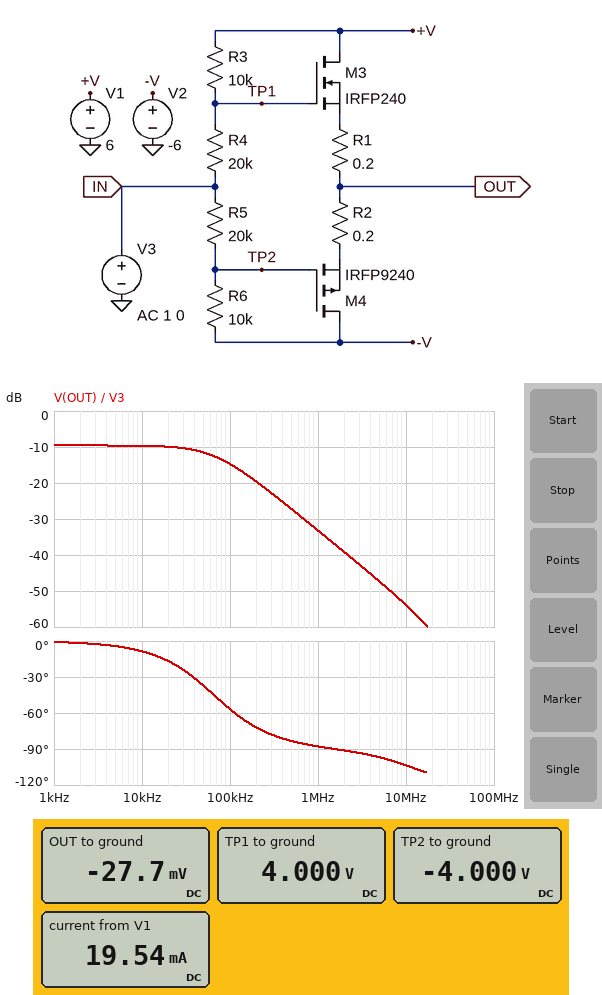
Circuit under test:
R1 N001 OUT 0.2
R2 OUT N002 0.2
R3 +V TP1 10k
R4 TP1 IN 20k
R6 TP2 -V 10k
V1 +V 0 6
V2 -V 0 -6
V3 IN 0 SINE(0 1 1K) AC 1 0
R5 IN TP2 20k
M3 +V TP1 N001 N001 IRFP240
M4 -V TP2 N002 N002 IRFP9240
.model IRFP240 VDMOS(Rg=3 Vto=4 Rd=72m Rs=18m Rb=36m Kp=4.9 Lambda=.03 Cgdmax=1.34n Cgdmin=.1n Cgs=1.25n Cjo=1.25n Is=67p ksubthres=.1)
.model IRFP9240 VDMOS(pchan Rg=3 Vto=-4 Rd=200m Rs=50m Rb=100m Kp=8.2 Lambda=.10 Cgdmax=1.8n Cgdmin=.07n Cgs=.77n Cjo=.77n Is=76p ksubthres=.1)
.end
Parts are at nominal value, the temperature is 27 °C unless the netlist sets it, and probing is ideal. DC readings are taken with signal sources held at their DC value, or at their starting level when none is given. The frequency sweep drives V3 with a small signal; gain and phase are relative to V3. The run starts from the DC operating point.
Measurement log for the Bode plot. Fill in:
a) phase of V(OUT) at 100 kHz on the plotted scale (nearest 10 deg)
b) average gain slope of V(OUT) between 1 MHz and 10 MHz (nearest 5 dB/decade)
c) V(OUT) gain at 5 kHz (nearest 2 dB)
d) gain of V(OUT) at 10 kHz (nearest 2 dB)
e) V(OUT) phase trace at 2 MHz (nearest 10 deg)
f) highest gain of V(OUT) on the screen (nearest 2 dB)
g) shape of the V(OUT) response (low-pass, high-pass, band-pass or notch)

-60 deg
-20 dB/decade
-10 dB
-10 dB
-90 deg
-10 dB
low-pass
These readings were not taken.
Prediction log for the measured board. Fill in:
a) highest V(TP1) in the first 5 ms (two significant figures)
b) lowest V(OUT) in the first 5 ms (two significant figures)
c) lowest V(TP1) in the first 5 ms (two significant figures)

4.3 V
-360 mV
3.7 V
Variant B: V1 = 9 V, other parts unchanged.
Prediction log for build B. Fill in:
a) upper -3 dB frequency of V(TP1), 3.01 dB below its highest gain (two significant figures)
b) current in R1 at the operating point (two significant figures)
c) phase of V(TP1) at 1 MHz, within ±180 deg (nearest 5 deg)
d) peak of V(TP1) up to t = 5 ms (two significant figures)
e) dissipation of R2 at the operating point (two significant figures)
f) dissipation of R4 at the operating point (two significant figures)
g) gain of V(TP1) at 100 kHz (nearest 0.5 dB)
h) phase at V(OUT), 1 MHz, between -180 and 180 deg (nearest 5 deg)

76 kHz
1.6 A
-85 deg
6.3 V
540 mW
1.8 mW
-14.0 dB
-85 deg
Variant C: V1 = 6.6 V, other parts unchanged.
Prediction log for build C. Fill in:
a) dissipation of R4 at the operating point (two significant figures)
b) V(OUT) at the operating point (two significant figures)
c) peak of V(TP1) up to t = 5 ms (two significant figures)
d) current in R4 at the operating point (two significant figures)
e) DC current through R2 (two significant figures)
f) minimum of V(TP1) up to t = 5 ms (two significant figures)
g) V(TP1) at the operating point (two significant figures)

970 µW
160 mV
4.7 V
220 µA
140 mA
4.1 V
4.4 V
